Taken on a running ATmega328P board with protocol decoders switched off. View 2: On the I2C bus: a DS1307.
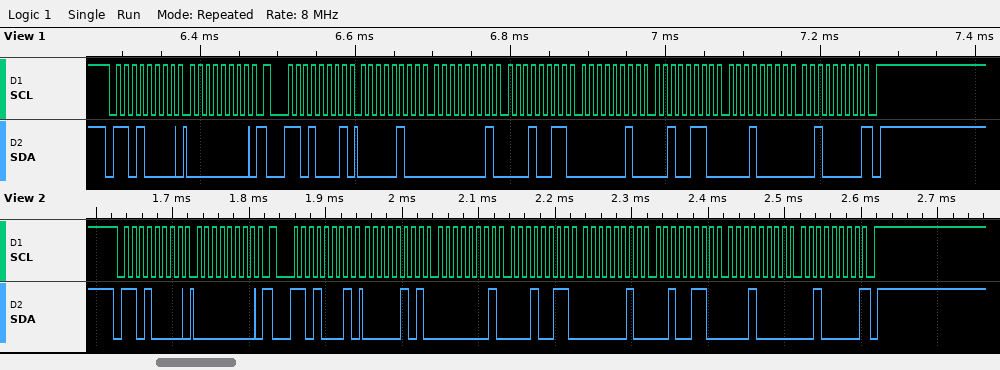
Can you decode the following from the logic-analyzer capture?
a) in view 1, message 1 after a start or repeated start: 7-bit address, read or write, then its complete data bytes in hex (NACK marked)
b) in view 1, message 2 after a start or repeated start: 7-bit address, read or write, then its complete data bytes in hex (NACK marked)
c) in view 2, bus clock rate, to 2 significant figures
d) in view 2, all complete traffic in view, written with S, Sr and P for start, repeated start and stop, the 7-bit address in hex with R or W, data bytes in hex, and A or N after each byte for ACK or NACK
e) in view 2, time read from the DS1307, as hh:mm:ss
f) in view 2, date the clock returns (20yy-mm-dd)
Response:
0x68 write: 00
0x68 read: 04 01 13 02 26 10 20 NACK
100 kHz
S 68W A 00 A Sr 68R A 05 A 01 A 13 A 02 A 26 A 10 A 20 N P
13:01:05
2020-10-26
